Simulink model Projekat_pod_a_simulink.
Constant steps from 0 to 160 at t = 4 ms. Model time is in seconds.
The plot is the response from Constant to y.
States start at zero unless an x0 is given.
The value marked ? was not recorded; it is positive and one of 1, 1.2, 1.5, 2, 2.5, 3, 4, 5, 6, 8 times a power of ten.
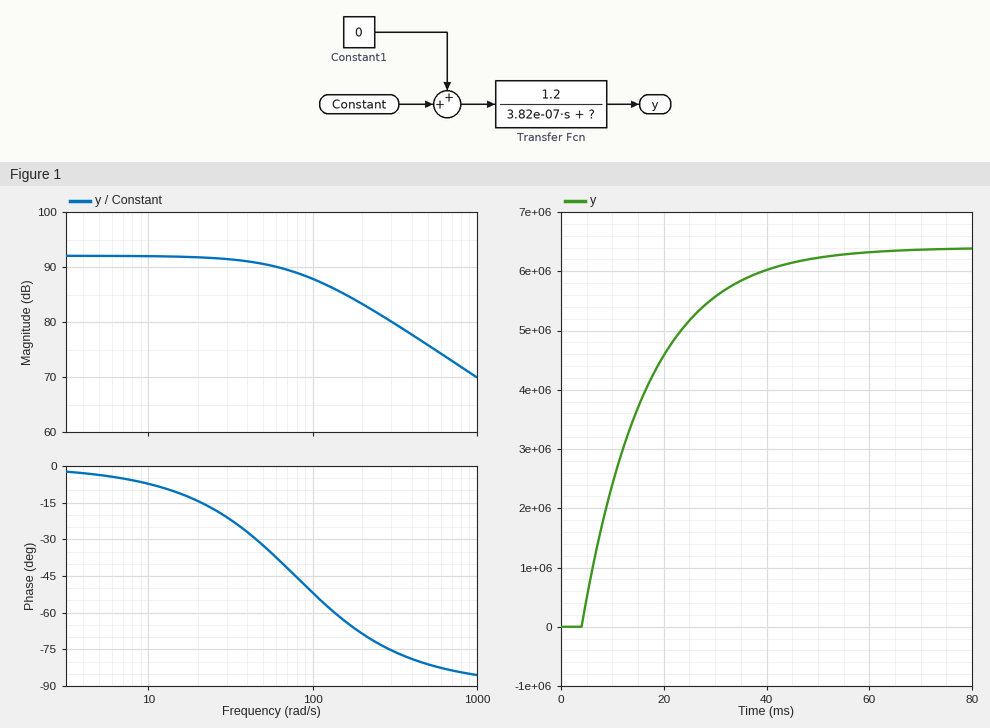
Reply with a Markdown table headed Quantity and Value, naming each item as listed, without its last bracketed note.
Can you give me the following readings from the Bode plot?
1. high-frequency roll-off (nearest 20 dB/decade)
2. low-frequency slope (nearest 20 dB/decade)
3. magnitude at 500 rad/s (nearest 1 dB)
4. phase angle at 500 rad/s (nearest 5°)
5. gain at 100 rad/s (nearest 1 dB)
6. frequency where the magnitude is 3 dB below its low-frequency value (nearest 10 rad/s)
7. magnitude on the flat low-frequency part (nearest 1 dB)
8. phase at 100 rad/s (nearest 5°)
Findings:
| Quantity | Value |
|---|---|
| high-frequency roll-off | -20 dB/decade |
| low-frequency slope | 0 dB/decade |
| magnitude at 500 rad/s | 76 dB |
| phase angle at 500 rad/s | -80° |
| gain at 100 rad/s | 88 dB |
| frequency where the magnitude is 3 dB below its low-frequency value | 80 rad/s |
| magnitude on the flat low-frequency part | 92 dB |
| phase at 100 rad/s | -50° |
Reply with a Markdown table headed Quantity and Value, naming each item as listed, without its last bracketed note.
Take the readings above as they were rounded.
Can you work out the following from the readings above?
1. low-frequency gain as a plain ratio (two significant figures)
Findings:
| Quantity | Value |
|---|---|
| low-frequency gain as a plain ratio | 40000 |
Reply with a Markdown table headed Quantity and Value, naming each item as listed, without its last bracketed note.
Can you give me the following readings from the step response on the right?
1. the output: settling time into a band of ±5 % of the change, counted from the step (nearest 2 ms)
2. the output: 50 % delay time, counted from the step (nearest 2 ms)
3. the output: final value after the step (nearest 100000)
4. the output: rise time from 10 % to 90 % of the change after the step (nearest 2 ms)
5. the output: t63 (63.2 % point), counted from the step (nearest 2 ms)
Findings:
| Quantity | Value |
|---|---|
| the output: settling time into a band of ±5 % of the change, counted from the step | 38 ms |
| the output: 50 % delay time, counted from the step | 8 ms |
| the output: final value after the step | 6400000 |
| the output: rise time from 10 % to 90 % of the change after the step | 28 ms |
| the output: t63 (63.2 % point), counted from the step | 12 ms |
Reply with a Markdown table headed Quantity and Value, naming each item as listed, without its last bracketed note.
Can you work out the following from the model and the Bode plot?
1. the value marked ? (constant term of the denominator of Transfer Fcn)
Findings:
| Quantity | Value |
|---|---|
| the value marked ? | 3e-05 |
